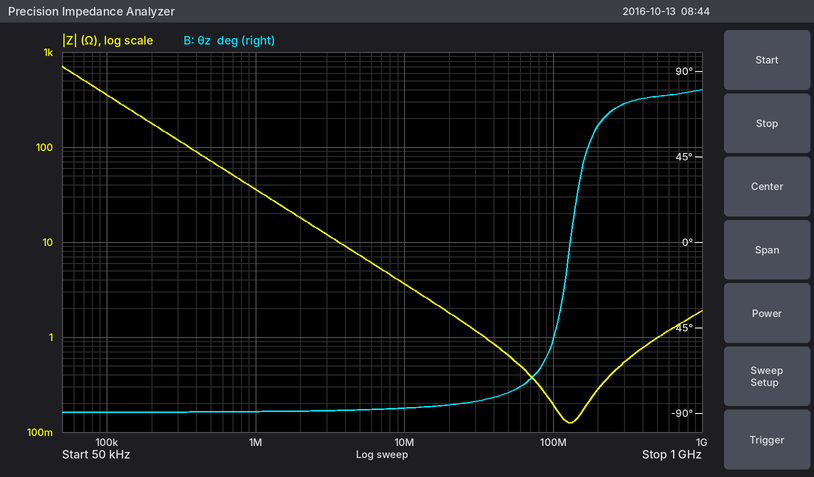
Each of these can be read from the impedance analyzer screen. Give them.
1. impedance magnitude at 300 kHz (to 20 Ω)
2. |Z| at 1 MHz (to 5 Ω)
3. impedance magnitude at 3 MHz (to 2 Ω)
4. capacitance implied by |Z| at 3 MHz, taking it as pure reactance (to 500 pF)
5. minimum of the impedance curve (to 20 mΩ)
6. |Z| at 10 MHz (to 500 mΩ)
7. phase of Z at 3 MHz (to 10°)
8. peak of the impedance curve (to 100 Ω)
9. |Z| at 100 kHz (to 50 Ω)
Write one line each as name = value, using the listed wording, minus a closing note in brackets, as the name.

impedance magnitude at 300 kHz = 120 Ω
|Z| at 1 MHz = 35 Ω
impedance magnitude at 3 MHz = 12 Ω
capacitance implied by |Z| at 3 MHz, taking it as pure reactance = 4.5 nF
minimum of the impedance curve = 120 mΩ
|Z| at 10 MHz = 3.5 Ω
phase of Z at 3 MHz = -90°
peak of the impedance curve = 700 Ω
|Z| at 100 kHz = 350 Ω
